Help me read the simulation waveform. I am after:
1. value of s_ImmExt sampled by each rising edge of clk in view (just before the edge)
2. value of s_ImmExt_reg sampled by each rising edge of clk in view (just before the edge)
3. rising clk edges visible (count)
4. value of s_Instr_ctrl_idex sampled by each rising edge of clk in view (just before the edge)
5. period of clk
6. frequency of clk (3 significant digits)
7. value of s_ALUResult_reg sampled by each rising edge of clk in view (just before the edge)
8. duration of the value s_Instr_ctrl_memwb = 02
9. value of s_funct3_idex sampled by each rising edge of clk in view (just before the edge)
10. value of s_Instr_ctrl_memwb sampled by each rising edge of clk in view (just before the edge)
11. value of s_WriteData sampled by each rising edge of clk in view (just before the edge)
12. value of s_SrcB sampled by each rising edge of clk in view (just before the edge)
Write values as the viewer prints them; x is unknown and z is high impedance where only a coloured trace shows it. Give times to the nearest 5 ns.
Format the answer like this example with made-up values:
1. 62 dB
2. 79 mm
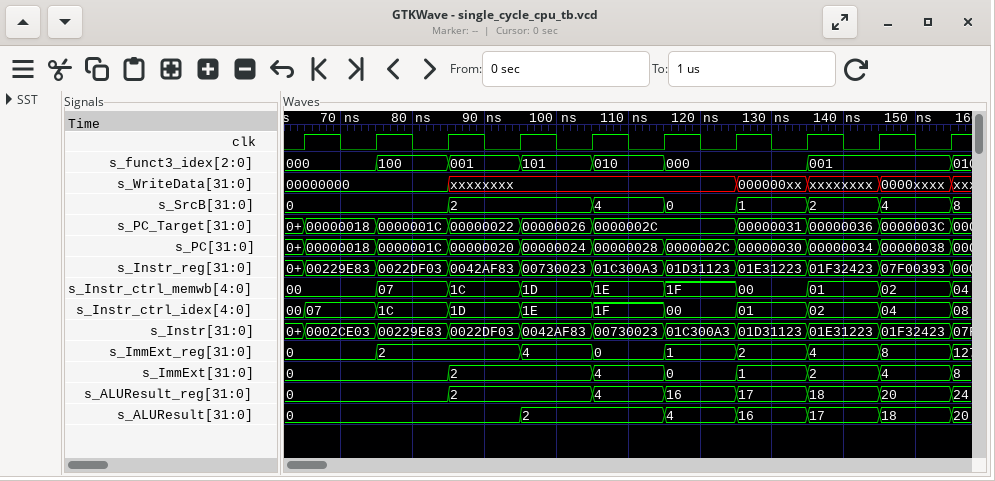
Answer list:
1. 0, 0, 0, 2, 2, 4, 0, 1, 2, 4
2. 0, 0, 2, 2, 4, 0, 1, 2, 4, 8
3. 10
4. 00, 07, 1C, 1D, 1E, 1F, 00, 01, 02, 04
5. 10 ns
6. 100 MHz
7. 0, 0, 0, 2, 2, 4, 16, 17, 18, 20
8. 10 ns
9. 000, 000, 100, 001, 101, 010, 000, 000, 001, 001
10. 00, 00, 07, 1C, 1D, 1E, 1F, 00, 01, 02
11. 00000000, 00000000, 00000000, xxxxxxxx, xxxxxxxx, xxxxxxxx, xxxxxxxx, 000000xx, xxxxxxxx, 0000xxxx
12. 0, 0, 0, 2, 2, 4, 0, 1, 2, 4
